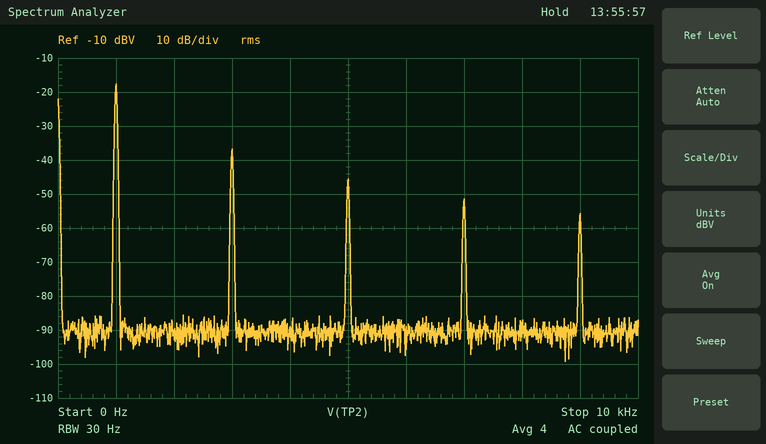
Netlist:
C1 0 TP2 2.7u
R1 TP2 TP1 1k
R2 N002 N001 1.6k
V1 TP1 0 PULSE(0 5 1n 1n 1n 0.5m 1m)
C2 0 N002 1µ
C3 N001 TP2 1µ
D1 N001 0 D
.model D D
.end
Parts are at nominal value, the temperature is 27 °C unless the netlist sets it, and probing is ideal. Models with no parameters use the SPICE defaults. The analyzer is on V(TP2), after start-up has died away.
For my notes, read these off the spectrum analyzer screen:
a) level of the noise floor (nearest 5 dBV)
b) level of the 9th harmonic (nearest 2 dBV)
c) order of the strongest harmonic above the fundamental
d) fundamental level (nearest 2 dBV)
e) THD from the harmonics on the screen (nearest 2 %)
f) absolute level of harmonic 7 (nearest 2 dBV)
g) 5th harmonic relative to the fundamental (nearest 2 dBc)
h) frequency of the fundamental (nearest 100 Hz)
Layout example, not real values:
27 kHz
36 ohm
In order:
-90 dBV
-56 dBV
3
-18 dBV
12 %
-52 dBV
-28 dBc
1.0 kHz
